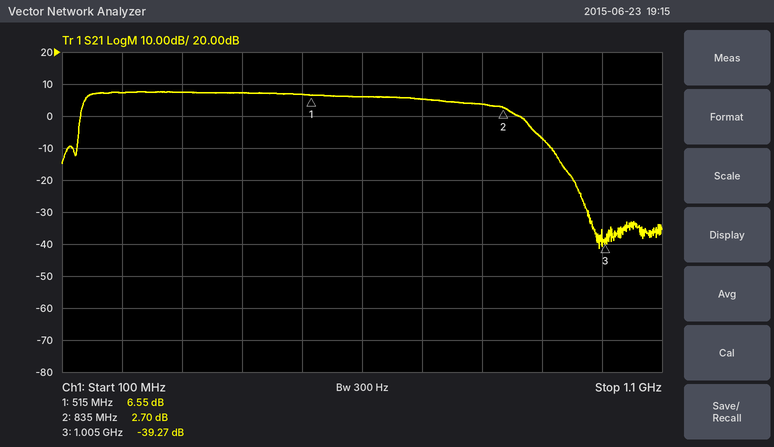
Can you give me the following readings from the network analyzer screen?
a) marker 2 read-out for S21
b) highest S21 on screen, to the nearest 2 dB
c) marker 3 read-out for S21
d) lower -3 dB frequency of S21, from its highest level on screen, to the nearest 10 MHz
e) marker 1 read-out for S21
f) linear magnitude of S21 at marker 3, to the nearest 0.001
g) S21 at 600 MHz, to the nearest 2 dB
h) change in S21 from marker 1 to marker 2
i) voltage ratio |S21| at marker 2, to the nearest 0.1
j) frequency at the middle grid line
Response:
2.70 dB
8 dB
-39.27 dB
140 MHz
6.55 dB
0.011
6 dB
-3.85 dB
1.4
600 MHz
